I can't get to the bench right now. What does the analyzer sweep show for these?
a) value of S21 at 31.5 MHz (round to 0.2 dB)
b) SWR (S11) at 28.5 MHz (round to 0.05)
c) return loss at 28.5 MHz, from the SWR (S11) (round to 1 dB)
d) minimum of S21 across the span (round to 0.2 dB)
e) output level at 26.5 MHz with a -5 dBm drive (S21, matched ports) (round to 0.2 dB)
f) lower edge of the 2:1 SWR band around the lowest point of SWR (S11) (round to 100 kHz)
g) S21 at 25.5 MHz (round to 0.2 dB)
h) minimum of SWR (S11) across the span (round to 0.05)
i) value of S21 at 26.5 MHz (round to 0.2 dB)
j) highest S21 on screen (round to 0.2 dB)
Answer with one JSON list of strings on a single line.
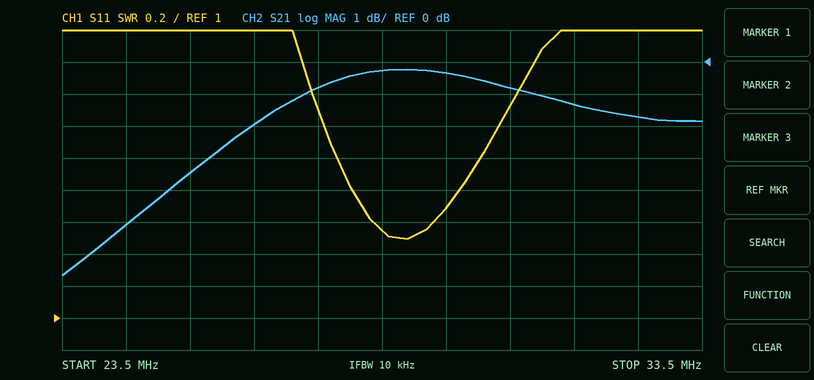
["-1.4 dB", "1.55", "13 dB", "-6.6 dB", "-7.0 dBm", "27.8 MHz", "-3.4 dB", "1.50", "-2.0 dB", "-0.2 dB"]
